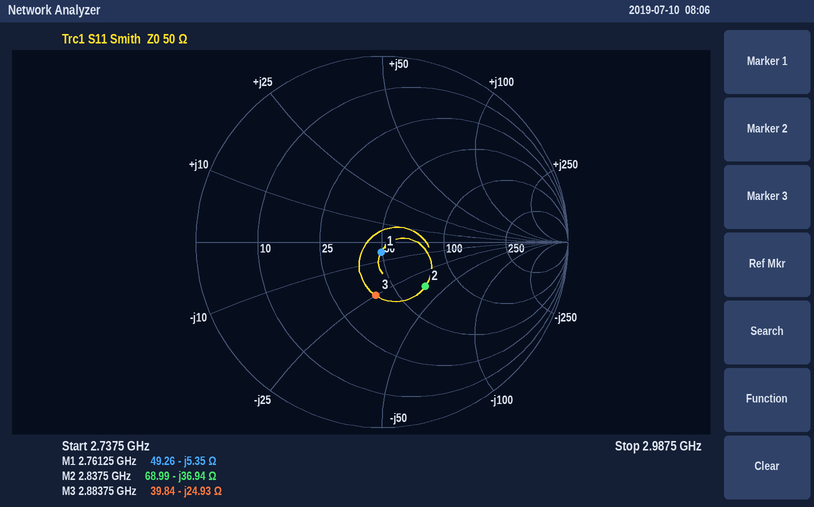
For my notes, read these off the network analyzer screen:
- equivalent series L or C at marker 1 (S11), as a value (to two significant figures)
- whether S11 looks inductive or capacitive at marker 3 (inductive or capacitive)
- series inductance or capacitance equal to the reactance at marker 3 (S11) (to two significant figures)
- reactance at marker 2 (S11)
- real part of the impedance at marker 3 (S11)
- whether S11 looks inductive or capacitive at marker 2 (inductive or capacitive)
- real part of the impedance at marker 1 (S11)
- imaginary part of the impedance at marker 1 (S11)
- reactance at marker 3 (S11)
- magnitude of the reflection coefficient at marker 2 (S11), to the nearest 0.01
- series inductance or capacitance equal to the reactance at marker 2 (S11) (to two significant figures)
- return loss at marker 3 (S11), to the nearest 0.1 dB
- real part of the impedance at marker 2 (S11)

11 pF
capacitive
2.2 pF
-36.94 Ω
39.84 Ω
capacitive
49.26 Ω
-5.35 Ω
-24.93 Ω
0.33
1.5 pF
10.8 dB
68.99 Ω
